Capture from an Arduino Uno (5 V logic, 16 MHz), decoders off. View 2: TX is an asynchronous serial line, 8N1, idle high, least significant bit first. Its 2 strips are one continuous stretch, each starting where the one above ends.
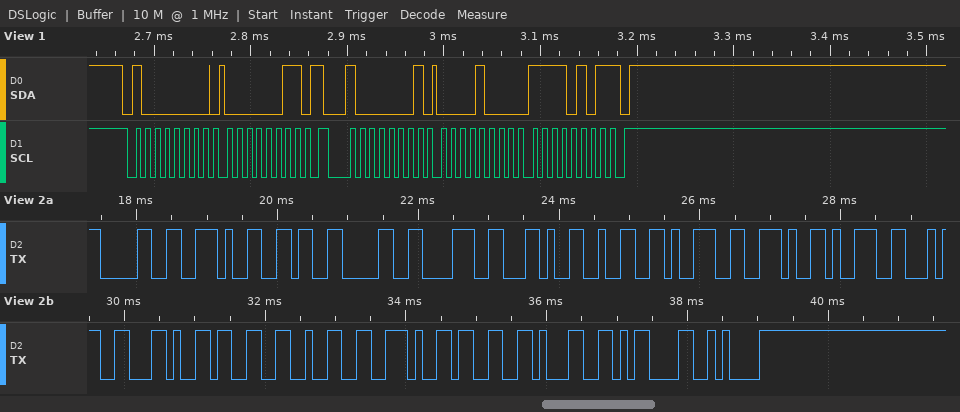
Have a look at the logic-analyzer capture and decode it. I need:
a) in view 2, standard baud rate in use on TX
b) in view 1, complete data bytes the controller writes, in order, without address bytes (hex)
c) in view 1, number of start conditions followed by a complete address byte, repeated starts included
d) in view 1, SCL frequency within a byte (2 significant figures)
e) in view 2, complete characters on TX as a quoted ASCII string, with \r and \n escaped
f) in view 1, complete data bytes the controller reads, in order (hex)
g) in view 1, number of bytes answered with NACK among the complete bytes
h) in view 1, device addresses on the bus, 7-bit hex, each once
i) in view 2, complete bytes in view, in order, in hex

9600 baud
03
2
100 kHz
"0.608,29.94,32.31\r\n"
08 F5
1
0x40
30 2E 36 30 38 2C 32 39 2E 39 34 2C 33 32 2E 33 31 0D 0A
